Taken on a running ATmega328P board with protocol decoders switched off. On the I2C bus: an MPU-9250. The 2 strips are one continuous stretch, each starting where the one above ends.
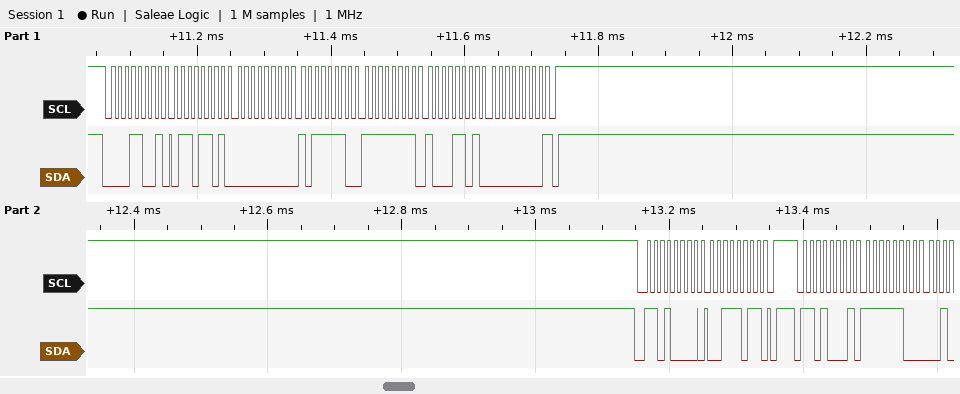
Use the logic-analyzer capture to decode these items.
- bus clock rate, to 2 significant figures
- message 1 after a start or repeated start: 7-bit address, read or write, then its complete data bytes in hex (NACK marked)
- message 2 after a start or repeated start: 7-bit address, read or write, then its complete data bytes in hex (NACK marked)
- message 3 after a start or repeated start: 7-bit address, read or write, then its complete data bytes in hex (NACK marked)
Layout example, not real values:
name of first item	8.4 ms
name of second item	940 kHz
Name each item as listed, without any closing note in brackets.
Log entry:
bus clock rate, to 2 significant figures	100 kHz
message 1 after a start or repeated start: 7-bit address, read or write, then its complete data bytes in hex	0x0C read: 6D 00 BE FF 8D 00 NACK
message 2 after a start or repeated start: 7-bit address, read or write, then its complete data bytes in hex	0x68 write: 3B
message 3 after a start or repeated start: 7-bit address, read or write, then its complete data bytes in hex	0x68 read: FC
